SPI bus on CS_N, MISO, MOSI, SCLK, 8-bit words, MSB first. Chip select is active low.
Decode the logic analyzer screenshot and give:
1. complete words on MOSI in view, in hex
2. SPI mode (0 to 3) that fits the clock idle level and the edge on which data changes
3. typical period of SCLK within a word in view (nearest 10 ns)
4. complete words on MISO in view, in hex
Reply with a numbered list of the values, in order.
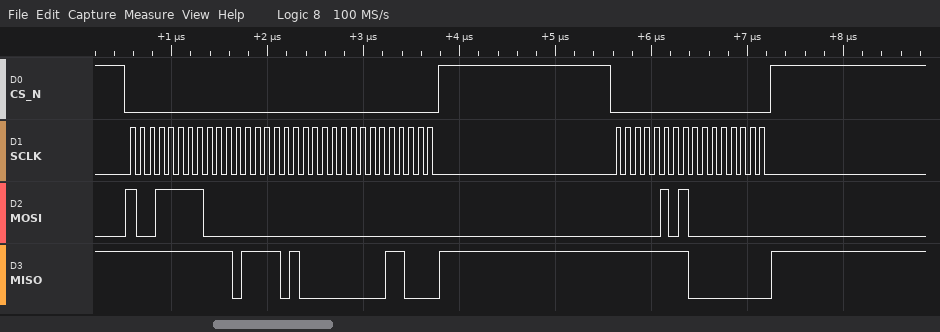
1. 9F, 00, 00, 00, 05, 00
2. 0
3. 100 ns
4. FF, EF, 40, 18, FF, 00
